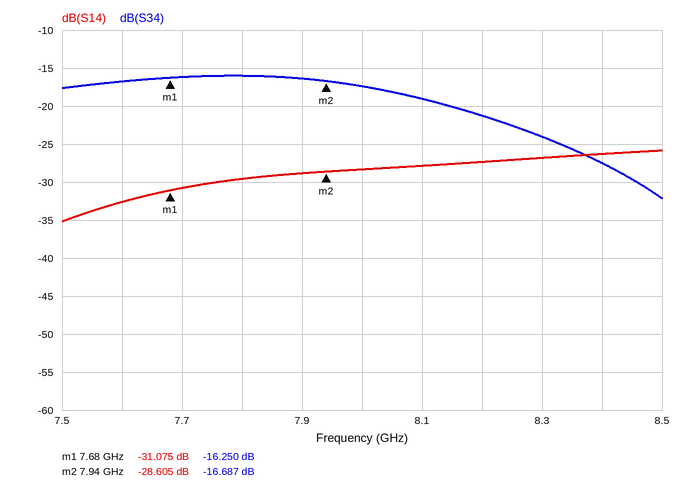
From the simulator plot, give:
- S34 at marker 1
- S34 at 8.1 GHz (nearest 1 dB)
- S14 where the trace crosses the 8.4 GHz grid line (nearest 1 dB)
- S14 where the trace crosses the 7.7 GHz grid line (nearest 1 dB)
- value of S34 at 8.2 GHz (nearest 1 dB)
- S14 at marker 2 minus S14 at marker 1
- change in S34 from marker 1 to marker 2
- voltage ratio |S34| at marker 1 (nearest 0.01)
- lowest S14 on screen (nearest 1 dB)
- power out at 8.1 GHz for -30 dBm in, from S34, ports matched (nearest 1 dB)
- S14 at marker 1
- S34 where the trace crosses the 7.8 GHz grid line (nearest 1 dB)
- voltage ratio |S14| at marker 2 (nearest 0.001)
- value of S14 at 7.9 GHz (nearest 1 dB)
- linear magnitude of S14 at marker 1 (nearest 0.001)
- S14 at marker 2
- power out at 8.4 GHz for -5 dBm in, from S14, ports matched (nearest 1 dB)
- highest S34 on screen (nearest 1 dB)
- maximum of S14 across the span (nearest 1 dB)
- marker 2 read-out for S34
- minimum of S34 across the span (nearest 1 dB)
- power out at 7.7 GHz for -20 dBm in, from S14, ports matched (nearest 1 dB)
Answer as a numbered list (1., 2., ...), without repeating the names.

1. -16.250 dB
2. -19 dB
3. -26 dB
4. -31 dB
5. -21 dB
6. 2.470 dB
7. -0.437 dB
8. 0.15
9. -35 dB
10. -49 dBm
11. -31.075 dB
12. -16 dB
13. 0.037
14. -29 dB
15. 0.028
16. -28.605 dB
17. -31 dBm
18. -16 dB
19. -26 dB
20. -16.687 dB
21. -32 dB
22. -51 dBm
